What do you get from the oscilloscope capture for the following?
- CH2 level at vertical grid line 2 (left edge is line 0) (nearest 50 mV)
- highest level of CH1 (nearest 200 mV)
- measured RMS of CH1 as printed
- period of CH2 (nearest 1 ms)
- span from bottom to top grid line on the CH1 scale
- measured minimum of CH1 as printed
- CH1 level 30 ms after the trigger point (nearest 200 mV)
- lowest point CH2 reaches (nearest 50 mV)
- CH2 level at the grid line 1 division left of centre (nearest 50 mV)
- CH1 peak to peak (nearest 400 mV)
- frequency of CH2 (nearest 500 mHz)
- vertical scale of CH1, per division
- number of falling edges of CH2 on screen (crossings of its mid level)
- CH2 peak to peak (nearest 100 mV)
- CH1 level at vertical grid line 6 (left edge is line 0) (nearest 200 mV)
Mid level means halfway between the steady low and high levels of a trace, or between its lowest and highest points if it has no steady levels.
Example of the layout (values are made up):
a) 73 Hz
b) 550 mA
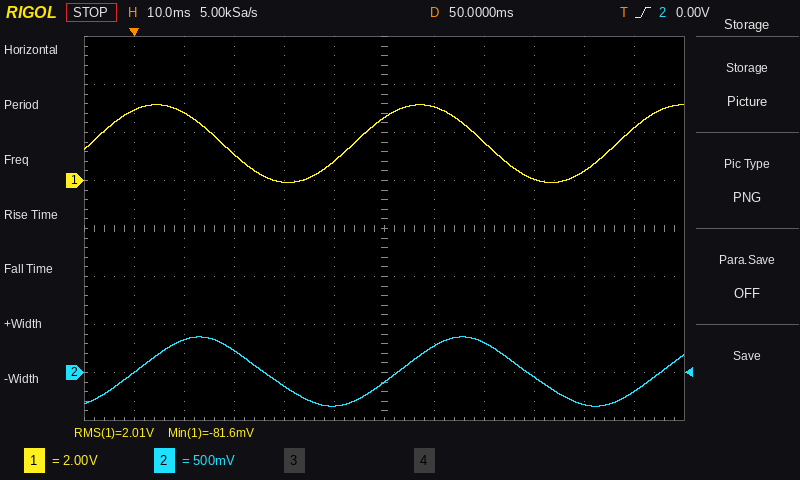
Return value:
a) 350 mV
b) 3.2 V
c) 2.01 V
d) 53 ms
e) 16 V
f) -81.6 mV
g) 0.0 V
h) -350 mV
i) -350 mV
j) 3.2 V
k) 19.0 Hz
l) 2 V
m) 2
n) 700 mV
o) 2.6 V
